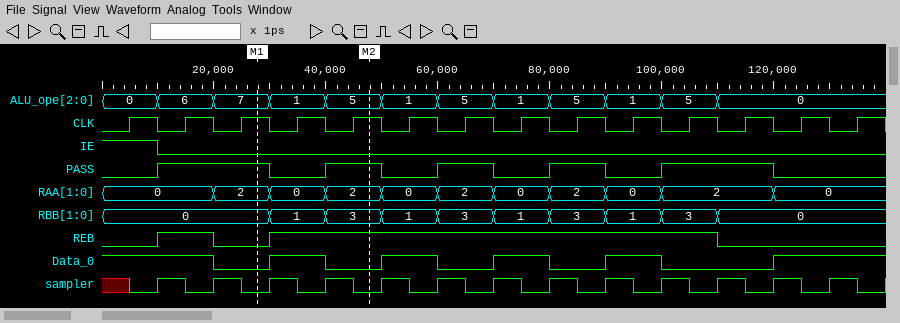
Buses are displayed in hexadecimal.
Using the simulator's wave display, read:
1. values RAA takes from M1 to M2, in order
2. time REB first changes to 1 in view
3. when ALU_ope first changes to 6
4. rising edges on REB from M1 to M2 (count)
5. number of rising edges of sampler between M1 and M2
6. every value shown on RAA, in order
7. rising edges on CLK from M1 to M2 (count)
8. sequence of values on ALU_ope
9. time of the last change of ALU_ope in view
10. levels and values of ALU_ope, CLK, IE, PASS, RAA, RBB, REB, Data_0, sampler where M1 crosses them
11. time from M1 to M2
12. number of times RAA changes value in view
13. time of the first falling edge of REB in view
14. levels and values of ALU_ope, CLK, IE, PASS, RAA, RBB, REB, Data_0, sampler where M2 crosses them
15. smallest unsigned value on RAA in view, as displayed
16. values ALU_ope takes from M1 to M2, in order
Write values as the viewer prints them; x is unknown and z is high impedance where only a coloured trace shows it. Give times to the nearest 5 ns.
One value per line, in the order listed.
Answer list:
2, 0, 2
10 ns
10 ns
1
2
0, 2, 0, 2, 0, 2, 0, 2, 0, 2, 0
2
0, 6, 7, 1, 5, 1, 5, 1, 5, 1, 5, 0
110 ns
ALU_ope=7, CLK=1, IE=0, PASS=1, RAA=2, RBB=0, REB=0, Data_0=0, sampler=0
20 ns
10
20 ns
ALU_ope=5, CLK=1, IE=0, PASS=1, RAA=2, RBB=3, REB=1, Data_0=0, sampler=0
0
7, 1, 5
